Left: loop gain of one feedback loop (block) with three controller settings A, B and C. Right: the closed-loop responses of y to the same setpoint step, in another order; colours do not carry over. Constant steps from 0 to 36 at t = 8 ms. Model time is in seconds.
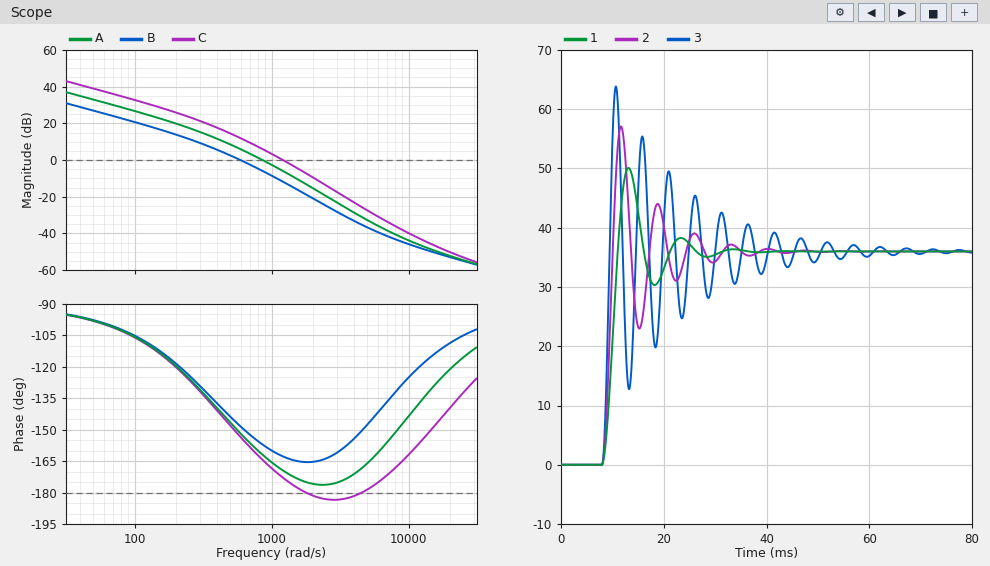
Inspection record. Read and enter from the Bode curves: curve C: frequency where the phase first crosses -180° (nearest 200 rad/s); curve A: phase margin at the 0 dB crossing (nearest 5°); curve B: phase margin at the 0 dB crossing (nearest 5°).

1800 rad/s
20°
30°
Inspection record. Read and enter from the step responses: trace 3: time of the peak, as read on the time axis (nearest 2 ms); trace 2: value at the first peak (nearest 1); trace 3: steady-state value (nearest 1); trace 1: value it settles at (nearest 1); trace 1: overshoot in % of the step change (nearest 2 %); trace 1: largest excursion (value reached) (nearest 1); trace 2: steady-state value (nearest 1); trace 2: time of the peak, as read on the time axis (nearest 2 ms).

10 ms
57
36
36
40 %
50
36
12 ms
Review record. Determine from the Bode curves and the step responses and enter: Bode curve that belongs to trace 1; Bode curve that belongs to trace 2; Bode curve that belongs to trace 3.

B
A
C
